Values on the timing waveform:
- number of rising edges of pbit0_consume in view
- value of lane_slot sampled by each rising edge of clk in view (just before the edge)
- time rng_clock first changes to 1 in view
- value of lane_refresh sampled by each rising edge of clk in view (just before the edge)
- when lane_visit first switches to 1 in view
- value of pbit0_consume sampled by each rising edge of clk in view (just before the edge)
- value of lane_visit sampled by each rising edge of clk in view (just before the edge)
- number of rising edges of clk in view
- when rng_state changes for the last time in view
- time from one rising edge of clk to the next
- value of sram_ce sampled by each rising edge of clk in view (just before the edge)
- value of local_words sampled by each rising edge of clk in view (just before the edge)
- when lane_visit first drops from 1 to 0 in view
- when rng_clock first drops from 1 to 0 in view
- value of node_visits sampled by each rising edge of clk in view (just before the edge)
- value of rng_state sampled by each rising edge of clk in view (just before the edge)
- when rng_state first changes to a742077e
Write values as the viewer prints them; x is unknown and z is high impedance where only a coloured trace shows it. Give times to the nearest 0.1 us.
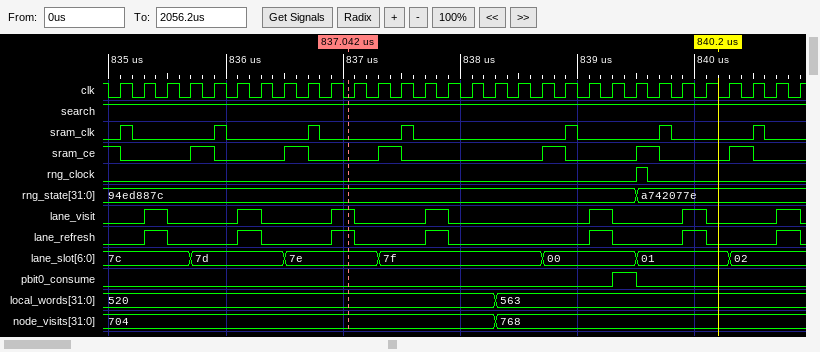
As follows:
1
7c, 7c, 7c, 7c, 7d, 7d, 7d, 7d, 7e, 7e, 7e, 7e, 7f, 7f, 7f, 7f, 7f, 7f, 7f, 00, 00, 00, 00, 01, 01, 01, 01, 02, 02, 02
839.5 us
0 0 1 0 0 0 1 0 0 0 1 0 0 0 1 0 0 0 0 0 0 1 0 0 0 1 0 0 0 1
835.3 us
0 0 0 0 0 0 0 0 0 0 0 0 0 0 0 0 0 0 0 0 0 0 1 0 0 0 0 0 0 0
0 0 1 0 0 0 1 0 0 0 1 0 0 0 1 0 0 0 0 0 0 1 0 0 0 1 0 0 0 1
30
839.5 us
0.2 us
1 0 0 0 1 0 0 0 1 0 0 0 1 0 0 0 0 0 0 1 0 0 0 1 0 0 0 1 0 0
520, 520, 520, 520, 520, 520, 520, 520, 520, 520, 520, 520, 520, 520, 520, 520, 520, 563, 563, 563, 563, 563, 563, 563, 563, 563, 563, 563, 563, 563
835.5 us
839.6 us
704, 704, 704, 704, 704, 704, 704, 704, 704, 704, 704, 704, 704, 704, 704, 704, 704, 768, 768, 768, 768, 768, 768, 768, 768, 768, 768, 768, 768, 768
94ed887c, 94ed887c, 94ed887c, 94ed887c, 94ed887c, 94ed887c, 94ed887c, 94ed887c, 94ed887c, 94ed887c, 94ed887c, 94ed887c, 94ed887c, 94ed887c, 94ed887c, 94ed887c, 94ed887c, 94ed887c, 94ed887c, 94ed887c, 94ed887c, 94ed887c, 94ed887c, a742077e, a742077e, a742077e, a742077e, a742077e, a742077e, a742077e
839.5 us
